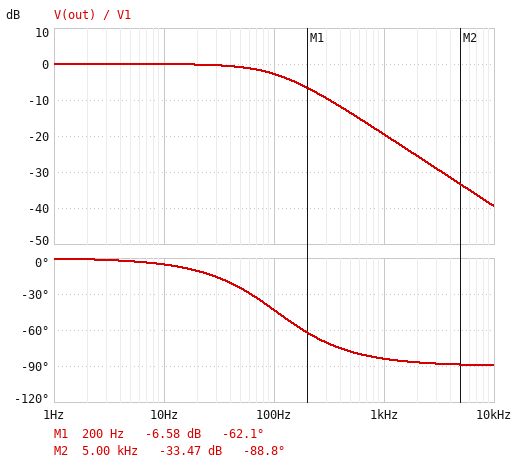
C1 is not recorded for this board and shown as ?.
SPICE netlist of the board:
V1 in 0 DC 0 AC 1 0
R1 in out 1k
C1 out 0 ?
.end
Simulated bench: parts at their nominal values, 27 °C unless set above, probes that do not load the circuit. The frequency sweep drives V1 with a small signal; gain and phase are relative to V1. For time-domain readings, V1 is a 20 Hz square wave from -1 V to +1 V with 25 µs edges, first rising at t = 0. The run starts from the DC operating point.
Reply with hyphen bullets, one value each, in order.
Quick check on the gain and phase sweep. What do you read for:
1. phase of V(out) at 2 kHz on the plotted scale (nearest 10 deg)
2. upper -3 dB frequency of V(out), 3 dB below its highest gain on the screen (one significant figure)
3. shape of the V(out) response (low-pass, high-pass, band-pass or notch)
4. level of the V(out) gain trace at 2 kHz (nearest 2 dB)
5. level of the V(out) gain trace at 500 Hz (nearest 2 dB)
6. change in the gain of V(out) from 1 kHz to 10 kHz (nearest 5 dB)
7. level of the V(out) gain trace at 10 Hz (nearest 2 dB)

- -90 deg
- 100 Hz
- low-pass
- -26 dB
- -14 dB
- -20 dB
- 0 dB
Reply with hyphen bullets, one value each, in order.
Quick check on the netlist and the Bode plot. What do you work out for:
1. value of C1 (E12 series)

- 1.5 µF
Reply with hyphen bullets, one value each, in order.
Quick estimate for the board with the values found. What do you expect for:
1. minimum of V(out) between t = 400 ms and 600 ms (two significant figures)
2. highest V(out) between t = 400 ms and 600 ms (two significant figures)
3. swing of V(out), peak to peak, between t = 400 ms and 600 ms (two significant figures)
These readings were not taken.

- -1.0 V
- 1.0 V
- 2.0 V
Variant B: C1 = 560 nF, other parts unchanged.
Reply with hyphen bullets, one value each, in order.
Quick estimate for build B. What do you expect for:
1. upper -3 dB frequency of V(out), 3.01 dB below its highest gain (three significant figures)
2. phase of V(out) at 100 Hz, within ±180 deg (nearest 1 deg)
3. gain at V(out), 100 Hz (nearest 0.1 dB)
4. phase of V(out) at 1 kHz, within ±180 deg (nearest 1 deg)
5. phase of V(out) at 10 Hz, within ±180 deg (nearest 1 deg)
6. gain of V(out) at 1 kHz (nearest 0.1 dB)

- 284 Hz
- -19 deg
- -0.5 dB
- -74 deg
- -2 deg
- -11.3 dB
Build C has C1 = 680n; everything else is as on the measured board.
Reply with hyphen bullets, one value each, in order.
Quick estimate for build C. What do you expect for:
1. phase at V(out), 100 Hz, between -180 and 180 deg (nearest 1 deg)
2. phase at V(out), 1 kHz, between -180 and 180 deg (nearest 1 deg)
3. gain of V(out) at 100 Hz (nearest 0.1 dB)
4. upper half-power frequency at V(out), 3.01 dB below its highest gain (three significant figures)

- -23 deg
- -77 deg
- -0.7 dB
- 234 Hz
